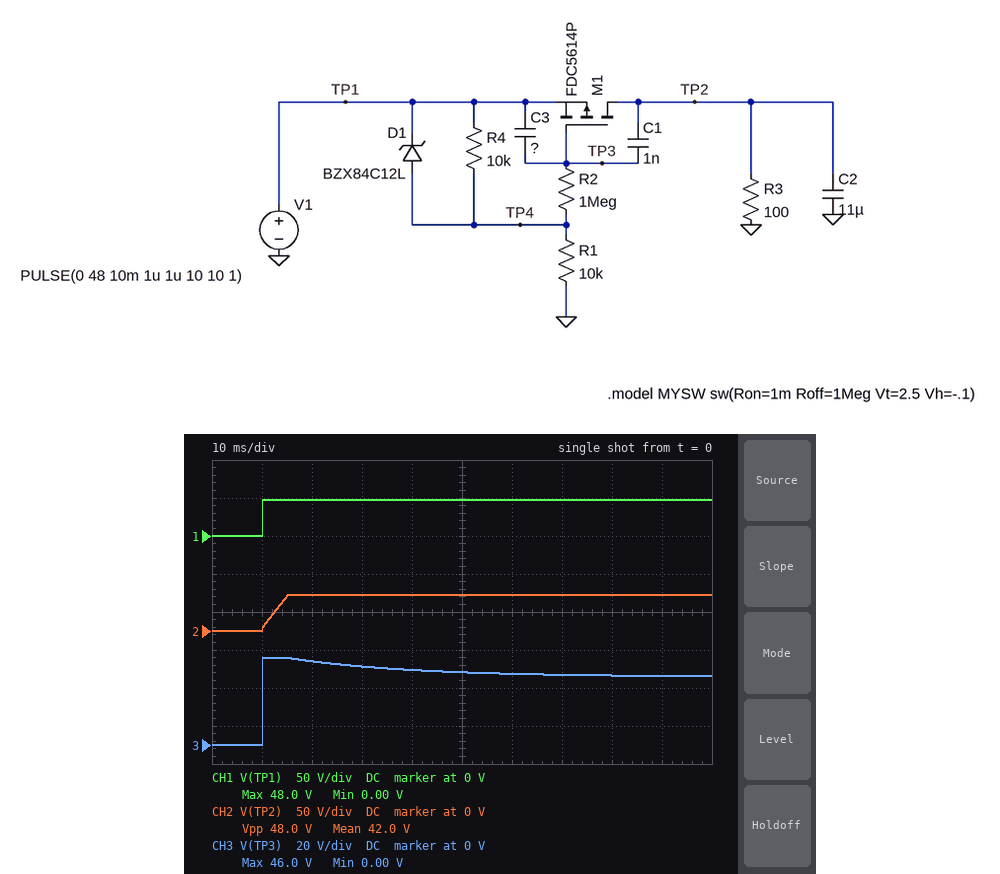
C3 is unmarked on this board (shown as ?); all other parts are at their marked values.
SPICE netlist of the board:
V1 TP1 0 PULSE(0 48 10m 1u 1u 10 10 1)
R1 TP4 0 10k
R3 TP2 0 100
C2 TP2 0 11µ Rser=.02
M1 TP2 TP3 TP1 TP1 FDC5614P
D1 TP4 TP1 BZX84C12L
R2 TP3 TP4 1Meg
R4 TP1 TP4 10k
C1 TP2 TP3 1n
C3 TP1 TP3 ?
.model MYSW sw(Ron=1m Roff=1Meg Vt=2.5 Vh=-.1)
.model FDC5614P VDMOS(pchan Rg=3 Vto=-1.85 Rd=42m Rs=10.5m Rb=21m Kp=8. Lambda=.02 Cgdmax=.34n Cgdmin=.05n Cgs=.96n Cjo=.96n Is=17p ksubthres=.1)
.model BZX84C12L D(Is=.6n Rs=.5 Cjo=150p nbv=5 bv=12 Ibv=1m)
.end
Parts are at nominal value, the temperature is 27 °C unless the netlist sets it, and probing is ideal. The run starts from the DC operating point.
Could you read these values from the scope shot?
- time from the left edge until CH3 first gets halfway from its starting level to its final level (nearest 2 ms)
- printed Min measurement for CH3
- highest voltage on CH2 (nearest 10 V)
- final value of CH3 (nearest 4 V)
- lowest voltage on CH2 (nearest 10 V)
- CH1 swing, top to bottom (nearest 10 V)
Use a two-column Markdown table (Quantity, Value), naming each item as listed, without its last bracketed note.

| Quantity | Value |
|---|---|
| time from the left edge until CH3 first gets halfway from its starting level to its final level | 10 ms |
| printed Min measurement for CH3 | 0.00 V |
| highest voltage on CH2 | 50 V |
| final value of CH3 | 36 V |
| lowest voltage on CH2 | 0 V |
| CH1 swing, top to bottom | 50 V |
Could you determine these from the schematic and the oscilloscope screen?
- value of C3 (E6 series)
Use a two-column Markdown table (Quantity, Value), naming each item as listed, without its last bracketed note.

| Quantity | Value |
|---|---|
| value of C3 | 22 nF |
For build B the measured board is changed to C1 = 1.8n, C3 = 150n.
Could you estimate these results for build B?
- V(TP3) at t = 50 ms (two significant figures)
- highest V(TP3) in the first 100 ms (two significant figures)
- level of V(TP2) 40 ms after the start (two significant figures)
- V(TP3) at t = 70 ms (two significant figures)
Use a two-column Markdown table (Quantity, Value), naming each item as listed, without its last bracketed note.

| Quantity | Value |
|---|---|
| V(TP3) at t = 50 ms | 45 V |
| highest V(TP3) in the first 100 ms | 47 V |
| level of V(TP2) 40 ms after the start | 41 V |
| V(TP3) at t = 70 ms | 44 V |
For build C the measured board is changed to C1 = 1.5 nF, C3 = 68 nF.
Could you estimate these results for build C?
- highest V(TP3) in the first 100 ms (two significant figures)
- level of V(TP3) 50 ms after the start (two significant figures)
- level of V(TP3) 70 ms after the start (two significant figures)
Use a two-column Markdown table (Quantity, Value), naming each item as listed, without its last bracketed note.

| Quantity | Value |
|---|---|
| highest V(TP3) in the first 100 ms | 47 V |
| level of V(TP3) 50 ms after the start | 43 V |
| level of V(TP3) 70 ms after the start | 41 V |
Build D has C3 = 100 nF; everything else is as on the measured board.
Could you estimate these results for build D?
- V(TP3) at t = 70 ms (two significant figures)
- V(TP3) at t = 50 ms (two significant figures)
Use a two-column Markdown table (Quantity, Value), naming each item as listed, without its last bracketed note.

| Quantity | Value |
|---|---|
| V(TP3) at t = 70 ms | 43 V |
| V(TP3) at t = 50 ms | 44 V |
